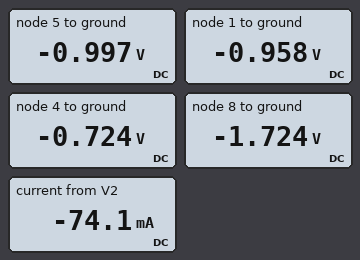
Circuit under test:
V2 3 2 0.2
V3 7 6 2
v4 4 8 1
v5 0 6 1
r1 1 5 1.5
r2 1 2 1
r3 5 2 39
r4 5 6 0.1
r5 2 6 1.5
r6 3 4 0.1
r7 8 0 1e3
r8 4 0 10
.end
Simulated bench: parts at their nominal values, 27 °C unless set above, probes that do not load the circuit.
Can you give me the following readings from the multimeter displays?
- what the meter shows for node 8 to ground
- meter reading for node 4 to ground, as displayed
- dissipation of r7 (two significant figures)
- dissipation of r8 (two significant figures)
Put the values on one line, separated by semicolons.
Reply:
-1.724 V; -0.724 V; 3.0 mW; 52 mW
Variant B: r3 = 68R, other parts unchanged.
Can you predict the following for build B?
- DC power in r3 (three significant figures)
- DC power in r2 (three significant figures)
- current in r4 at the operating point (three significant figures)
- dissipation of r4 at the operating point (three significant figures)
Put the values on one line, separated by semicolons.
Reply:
65.5 µW; 713 µW; 27.7 mA; 76.6 µW
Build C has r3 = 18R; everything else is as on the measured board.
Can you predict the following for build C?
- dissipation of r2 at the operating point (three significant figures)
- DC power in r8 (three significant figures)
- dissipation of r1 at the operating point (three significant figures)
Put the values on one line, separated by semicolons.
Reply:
664 µW; 52.6 mW; 996 µW
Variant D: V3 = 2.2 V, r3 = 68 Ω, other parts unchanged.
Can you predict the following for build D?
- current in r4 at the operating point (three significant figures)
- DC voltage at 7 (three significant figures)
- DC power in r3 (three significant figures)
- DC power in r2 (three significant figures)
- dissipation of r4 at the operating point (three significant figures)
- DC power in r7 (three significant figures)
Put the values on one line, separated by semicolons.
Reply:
27.7 mA; 1.20 V; 65.5 µW; 713 µW; 76.6 µW; 2.97 mW
